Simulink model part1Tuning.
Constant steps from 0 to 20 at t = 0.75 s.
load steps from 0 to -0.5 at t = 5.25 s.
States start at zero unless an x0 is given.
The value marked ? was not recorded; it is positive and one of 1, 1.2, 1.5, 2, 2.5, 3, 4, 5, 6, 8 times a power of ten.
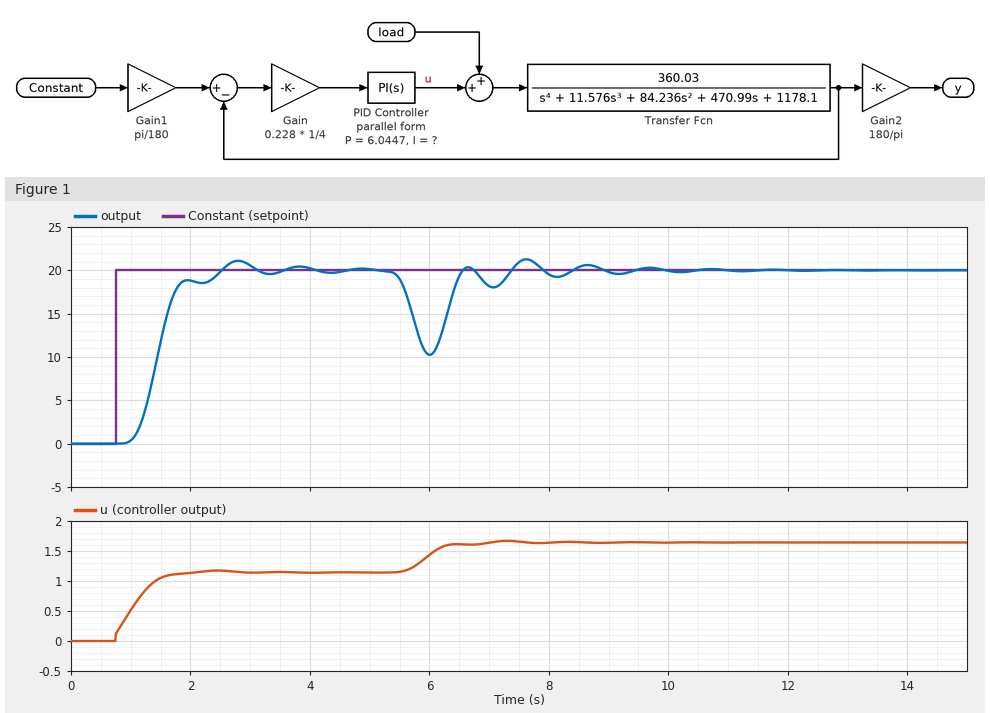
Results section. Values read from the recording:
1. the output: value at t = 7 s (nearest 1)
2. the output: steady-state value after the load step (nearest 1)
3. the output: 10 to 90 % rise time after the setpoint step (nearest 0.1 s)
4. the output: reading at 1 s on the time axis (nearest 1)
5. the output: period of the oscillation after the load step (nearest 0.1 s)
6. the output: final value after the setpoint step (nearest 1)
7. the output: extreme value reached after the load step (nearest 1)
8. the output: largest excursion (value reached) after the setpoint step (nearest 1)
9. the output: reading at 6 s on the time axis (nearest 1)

18
20
0.6 s
0
1.1 s
20
10
21
10
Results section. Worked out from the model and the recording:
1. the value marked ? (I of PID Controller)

80
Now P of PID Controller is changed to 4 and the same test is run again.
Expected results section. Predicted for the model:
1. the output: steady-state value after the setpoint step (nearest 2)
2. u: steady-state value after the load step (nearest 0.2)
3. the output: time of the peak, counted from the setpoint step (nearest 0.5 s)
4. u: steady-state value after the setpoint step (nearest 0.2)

20
1.6
2.0 s
1.2
